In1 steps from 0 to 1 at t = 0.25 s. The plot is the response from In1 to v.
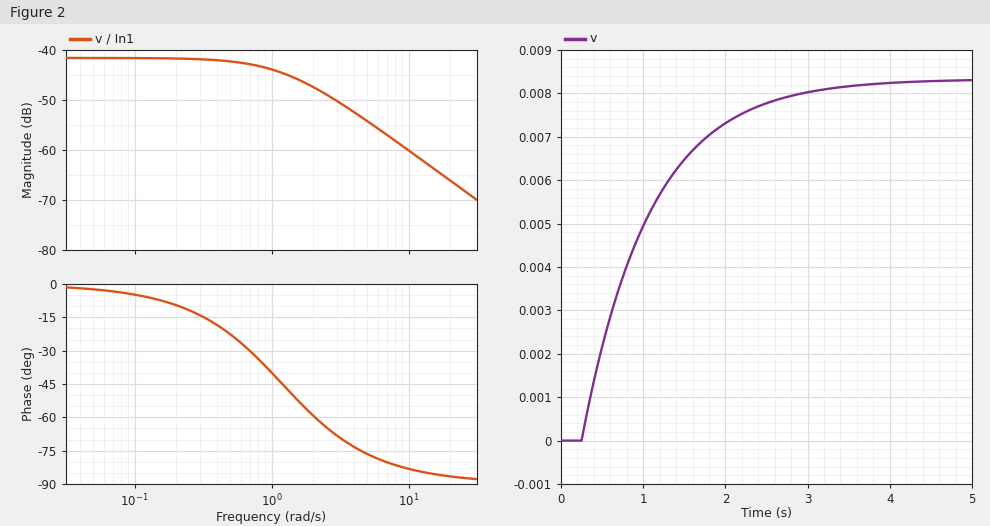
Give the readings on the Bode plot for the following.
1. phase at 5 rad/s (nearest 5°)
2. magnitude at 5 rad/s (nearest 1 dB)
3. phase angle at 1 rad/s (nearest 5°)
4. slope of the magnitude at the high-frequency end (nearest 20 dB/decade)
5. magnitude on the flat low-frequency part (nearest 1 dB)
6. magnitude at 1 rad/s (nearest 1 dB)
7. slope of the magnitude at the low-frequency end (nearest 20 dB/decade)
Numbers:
-75°
-54 dB
-40°
-20 dB/decade
-42 dB
-44 dB
0 dB/decade
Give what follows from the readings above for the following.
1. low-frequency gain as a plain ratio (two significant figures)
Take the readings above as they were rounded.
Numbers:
0.0079
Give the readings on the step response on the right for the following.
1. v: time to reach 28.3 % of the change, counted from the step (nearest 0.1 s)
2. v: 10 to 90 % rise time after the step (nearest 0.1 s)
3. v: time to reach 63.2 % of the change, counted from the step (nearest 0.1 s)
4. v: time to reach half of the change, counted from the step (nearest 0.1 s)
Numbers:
0.3 s
1.8 s
0.8 s
0.6 s
